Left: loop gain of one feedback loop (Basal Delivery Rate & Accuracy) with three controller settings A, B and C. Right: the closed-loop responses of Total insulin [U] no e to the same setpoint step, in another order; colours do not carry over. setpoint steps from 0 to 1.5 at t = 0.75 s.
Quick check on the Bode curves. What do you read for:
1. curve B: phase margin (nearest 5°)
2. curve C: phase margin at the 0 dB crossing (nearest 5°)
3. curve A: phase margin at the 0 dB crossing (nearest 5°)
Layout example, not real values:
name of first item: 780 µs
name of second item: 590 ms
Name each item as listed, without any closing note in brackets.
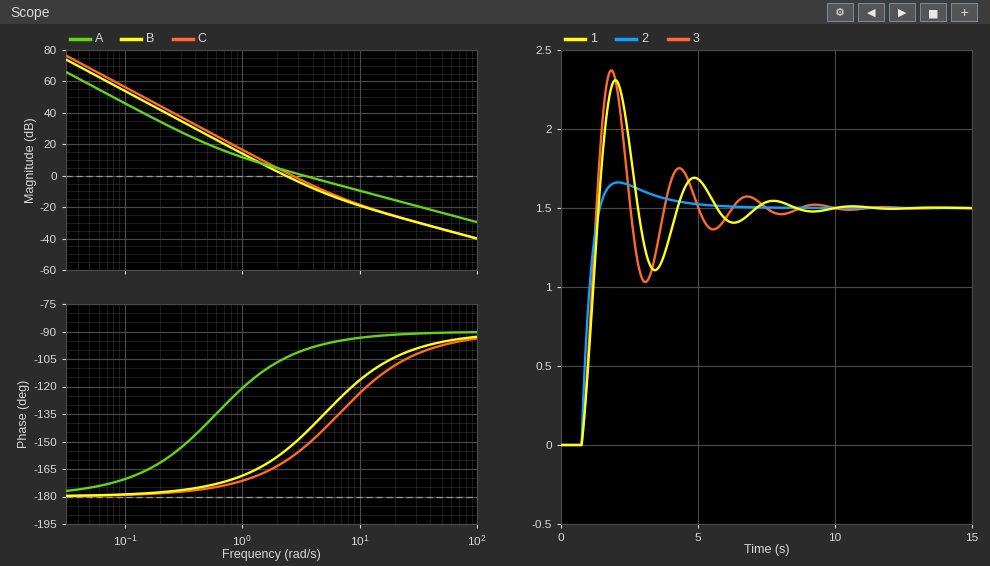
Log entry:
curve B: phase margin: 25°
curve C: phase margin at the 0 dB crossing: 20°
curve A: phase margin at the 0 dB crossing: 80°
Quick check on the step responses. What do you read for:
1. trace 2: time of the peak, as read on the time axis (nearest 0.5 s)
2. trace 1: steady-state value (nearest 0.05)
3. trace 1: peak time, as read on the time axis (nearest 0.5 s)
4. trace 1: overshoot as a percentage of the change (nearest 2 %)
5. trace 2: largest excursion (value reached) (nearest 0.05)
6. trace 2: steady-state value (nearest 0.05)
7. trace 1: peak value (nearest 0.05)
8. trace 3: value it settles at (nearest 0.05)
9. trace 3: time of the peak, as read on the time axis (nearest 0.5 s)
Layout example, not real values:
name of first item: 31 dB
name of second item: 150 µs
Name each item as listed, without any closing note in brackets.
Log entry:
trace 2: time of the peak, as read on the time axis: 2.0 s
trace 1: steady-state value: 1.50
trace 1: peak time, as read on the time axis: 2.0 s
trace 1: overshoot as a percentage of the change: 54 %
trace 2: largest excursion (value reached): 1.65
trace 2: steady-state value: 1.50
trace 1: peak value: 2.30
trace 3: value it settles at: 1.50
trace 3: time of the peak, as read on the time axis: 2.0 s
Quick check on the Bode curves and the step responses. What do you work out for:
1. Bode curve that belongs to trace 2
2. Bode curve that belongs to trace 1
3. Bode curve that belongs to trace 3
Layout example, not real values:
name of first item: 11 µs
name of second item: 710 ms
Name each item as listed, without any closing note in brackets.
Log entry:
Bode curve that belongs to trace 2: A
Bode curve that belongs to trace 1: B
Bode curve that belongs to trace 3: C
